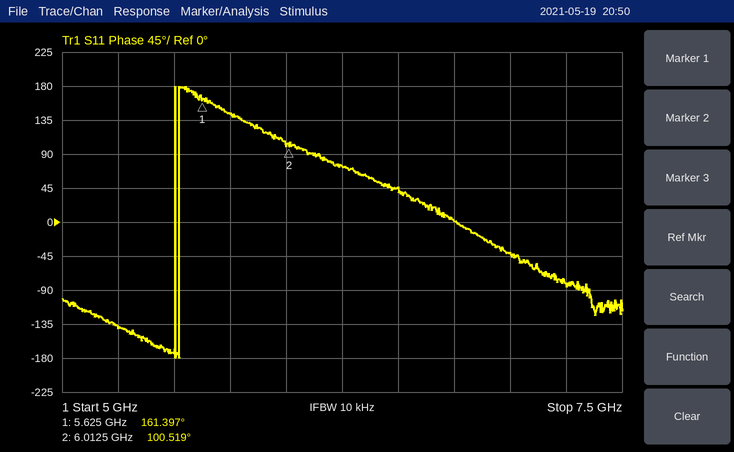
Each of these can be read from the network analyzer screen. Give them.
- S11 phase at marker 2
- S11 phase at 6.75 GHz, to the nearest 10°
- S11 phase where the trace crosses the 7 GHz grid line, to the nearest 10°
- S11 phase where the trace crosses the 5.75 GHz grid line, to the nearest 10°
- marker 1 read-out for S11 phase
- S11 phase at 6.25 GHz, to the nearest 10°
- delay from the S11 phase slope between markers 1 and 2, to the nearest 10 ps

100.519°
0°
-40°
140°
161.397°
70°
440 ps
